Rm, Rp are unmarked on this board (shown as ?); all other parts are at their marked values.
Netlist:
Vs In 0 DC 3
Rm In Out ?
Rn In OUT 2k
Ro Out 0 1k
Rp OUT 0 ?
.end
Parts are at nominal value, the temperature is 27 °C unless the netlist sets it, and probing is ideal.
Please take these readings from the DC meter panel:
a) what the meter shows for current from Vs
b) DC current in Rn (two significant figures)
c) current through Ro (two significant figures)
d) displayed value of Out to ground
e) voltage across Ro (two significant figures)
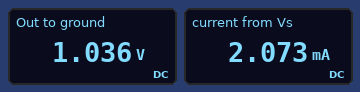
2.073 mA
980 µA
1.0 mA
1.036 V
1.0 V
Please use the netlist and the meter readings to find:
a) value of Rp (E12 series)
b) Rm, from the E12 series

1 kΩ
1.8 kΩ
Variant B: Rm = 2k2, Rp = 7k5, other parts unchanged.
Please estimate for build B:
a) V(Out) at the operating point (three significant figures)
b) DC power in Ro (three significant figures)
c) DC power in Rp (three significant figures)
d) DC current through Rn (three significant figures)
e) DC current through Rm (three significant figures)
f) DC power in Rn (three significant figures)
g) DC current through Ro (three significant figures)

1.37 V
1.88 mW
251 µW
814 µA
740 µA
1.33 mW
1.37 mA
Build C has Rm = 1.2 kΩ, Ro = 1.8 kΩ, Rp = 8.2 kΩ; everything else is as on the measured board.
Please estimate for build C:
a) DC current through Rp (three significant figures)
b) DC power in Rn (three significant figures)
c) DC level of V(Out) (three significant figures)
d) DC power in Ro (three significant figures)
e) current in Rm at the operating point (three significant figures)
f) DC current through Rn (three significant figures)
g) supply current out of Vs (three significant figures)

243 µA
511 µW
1.99 V
2.20 mW
842 µA
505 µA
1.35 mA
